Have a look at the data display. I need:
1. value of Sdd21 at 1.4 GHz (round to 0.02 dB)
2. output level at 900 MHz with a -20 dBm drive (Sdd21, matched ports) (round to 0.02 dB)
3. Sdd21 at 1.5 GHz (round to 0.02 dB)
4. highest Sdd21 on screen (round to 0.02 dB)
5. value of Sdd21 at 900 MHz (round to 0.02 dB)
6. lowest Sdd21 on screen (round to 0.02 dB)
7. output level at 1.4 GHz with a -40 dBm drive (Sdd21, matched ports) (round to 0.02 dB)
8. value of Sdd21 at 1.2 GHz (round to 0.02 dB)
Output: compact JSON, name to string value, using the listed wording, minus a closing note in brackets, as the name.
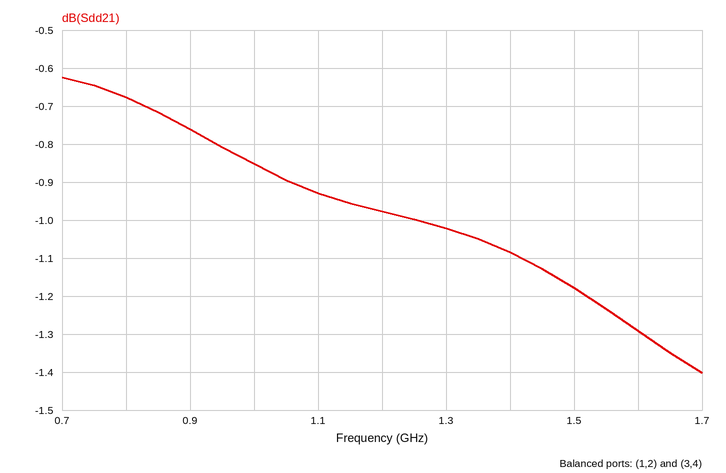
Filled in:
{"value of Sdd21 at 1.4 GHz": "-1.08 dB", "output level at 900 MHz with a -20 dBm drive (Sdd21, matched ports)": "-20.76 dBm", "Sdd21 at 1.5 GHz": "-1.18 dB", "highest Sdd21 on screen": "-0.62 dB", "value of Sdd21 at 900 MHz": "-0.76 dB", "lowest Sdd21 on screen": "-1.40 dB", "output level at 1.4 GHz with a -40 dBm drive (Sdd21, matched ports)": "-41.08 dBm", "value of Sdd21 at 1.2 GHz": "-0.98 dB"}
